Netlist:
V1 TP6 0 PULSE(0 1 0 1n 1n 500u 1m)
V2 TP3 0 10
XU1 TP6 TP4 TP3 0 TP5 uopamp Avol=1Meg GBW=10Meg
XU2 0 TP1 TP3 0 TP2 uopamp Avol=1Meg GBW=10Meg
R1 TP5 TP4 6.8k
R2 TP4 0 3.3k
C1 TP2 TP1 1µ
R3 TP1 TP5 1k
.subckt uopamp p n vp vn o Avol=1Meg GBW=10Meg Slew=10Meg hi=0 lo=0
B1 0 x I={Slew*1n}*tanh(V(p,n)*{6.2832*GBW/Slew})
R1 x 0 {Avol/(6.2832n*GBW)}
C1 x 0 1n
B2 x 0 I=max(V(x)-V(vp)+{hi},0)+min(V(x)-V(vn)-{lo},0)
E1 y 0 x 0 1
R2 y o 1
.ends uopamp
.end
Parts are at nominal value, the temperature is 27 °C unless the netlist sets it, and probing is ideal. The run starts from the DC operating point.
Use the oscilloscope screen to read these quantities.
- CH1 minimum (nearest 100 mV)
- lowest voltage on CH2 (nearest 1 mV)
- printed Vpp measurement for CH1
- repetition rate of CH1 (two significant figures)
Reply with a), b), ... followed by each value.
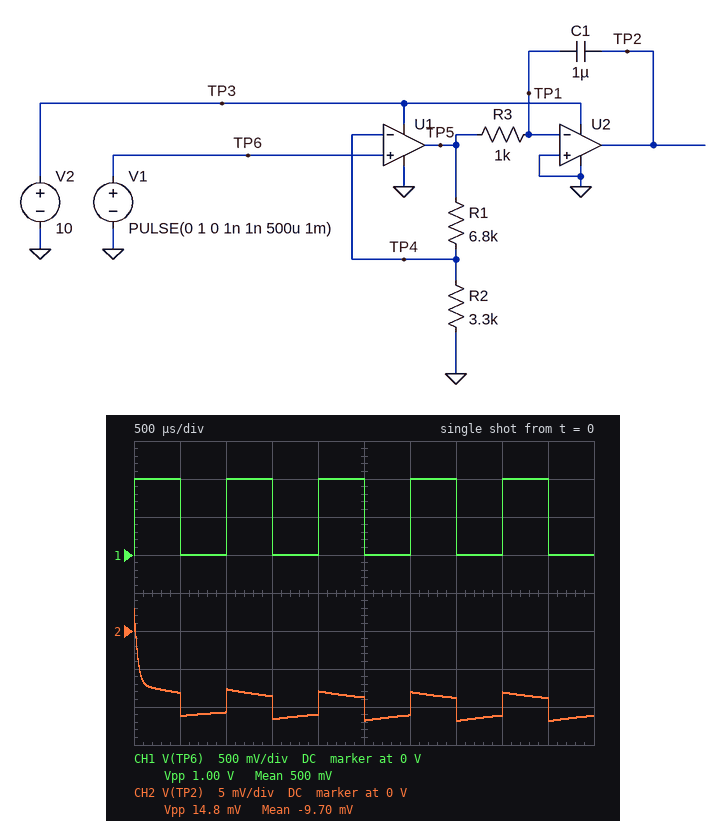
a) 0 V
b) -12 mV
c) 1.00 V
d) 1.0 kHz
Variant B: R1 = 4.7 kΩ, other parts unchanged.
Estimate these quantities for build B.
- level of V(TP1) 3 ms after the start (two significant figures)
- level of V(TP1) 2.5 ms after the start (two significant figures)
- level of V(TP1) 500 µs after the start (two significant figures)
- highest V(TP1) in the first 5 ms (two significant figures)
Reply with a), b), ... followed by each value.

a) 870 mV
b) 1.4 V
c) 950 mV
d) 1.5 V
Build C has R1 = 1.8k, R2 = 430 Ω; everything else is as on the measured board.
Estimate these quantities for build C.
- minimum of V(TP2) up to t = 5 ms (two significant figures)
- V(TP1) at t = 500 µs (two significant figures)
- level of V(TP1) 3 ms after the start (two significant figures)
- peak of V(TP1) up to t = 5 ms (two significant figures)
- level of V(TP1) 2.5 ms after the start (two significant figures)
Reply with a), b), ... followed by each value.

a) -13 mV
b) 2.0 V
c) 1.9 V
d) 3.2 V
e) 3.1 V
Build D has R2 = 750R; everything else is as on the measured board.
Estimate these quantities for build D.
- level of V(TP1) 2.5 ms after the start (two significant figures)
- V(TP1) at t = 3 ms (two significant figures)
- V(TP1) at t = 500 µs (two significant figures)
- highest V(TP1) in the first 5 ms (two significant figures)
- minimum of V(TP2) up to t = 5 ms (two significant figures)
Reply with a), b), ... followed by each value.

a) 5.9 V
b) 3.6 V
c) 3.9 V
d) 6.2 V
e) -16 mV
